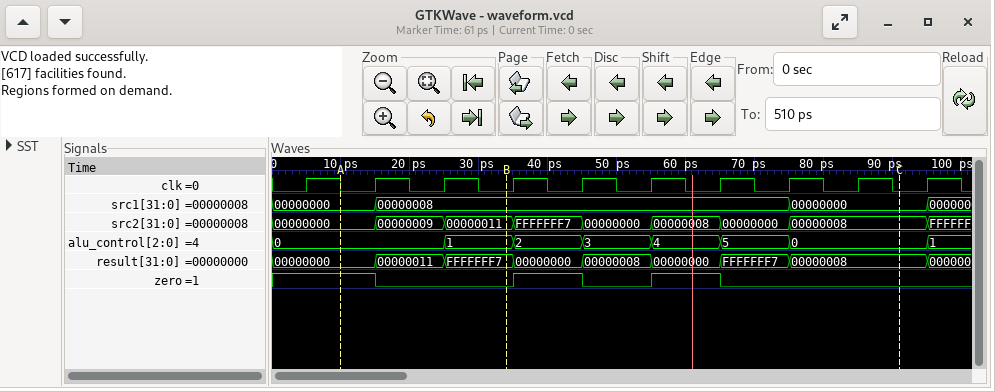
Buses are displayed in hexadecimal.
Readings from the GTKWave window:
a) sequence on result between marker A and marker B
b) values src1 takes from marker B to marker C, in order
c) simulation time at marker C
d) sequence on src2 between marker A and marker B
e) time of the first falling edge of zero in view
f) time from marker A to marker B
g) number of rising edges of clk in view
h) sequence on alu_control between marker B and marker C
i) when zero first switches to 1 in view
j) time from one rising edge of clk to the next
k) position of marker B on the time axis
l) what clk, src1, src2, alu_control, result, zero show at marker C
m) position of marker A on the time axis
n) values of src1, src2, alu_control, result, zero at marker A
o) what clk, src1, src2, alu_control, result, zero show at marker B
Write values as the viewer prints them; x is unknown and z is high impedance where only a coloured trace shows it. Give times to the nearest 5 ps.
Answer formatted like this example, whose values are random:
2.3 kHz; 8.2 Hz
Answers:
00000000, 00000011, FFFFFFF7; 00000008, 00000000; 90 ps; 00000000, 00000009, 00000011; 15 ps; 25 ps; 10; 1, 2, 3, 4, 5, 0; 35 ps; 10 ps; 35 ps; clk=0, src1=00000000, src2=00000008, alu_control=0, result=00000008, zero=0; 10 ps; src1=00000000, src2=00000000, alu_control=0, result=00000000, zero=1; clk=0, src1=00000008, src2=00000011, alu_control=1, result=FFFFFFF7, zero=0
